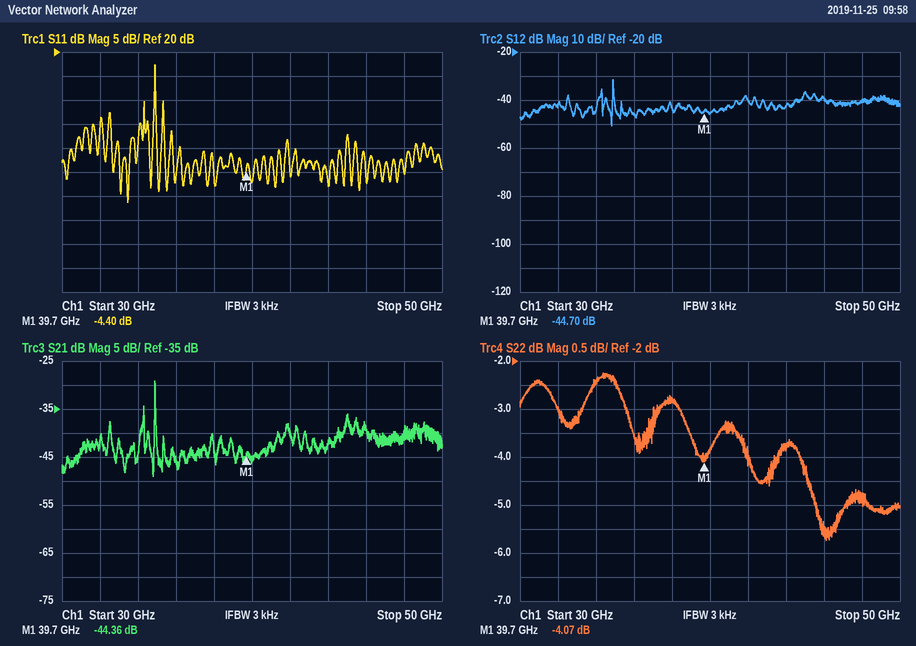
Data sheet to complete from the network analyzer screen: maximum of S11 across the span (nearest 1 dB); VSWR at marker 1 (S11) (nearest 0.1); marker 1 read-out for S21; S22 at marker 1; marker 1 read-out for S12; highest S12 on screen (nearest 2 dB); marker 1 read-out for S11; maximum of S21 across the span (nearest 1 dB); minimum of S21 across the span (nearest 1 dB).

17 dB
4.0
-44.36 dB
-4.07 dB
-44.70 dB
-32 dB
-4.40 dB
-29 dB
-49 dB
